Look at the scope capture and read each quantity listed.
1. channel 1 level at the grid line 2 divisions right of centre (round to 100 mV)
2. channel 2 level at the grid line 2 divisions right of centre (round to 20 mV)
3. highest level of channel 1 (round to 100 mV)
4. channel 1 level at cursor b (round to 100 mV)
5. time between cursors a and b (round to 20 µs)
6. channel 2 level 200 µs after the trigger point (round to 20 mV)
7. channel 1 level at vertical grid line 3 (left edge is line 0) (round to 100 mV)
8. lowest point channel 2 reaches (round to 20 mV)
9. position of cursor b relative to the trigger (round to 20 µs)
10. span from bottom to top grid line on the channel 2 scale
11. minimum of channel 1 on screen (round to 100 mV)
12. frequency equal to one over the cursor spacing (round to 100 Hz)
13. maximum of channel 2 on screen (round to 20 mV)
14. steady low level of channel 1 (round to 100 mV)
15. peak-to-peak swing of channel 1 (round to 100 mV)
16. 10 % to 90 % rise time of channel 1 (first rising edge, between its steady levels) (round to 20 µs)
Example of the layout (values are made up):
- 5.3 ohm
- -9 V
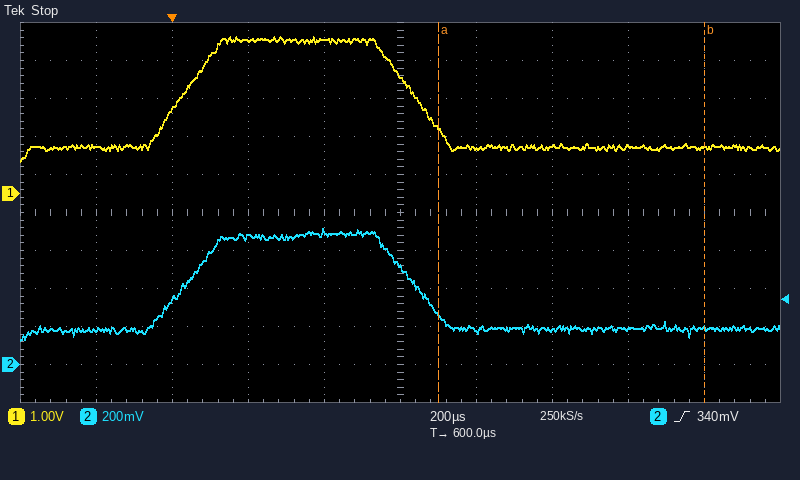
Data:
- 1.2 V
- 180 mV
- 4.1 V
- 1.2 V
- 700 µs
- 660 mV
- 4.0 V
- 120 mV
- +1.40 ms
- 2 V
- 800 mV
- 1.4 kHz
- 720 mV
- 1.2 V
- 3.3 V
- 160 µs
